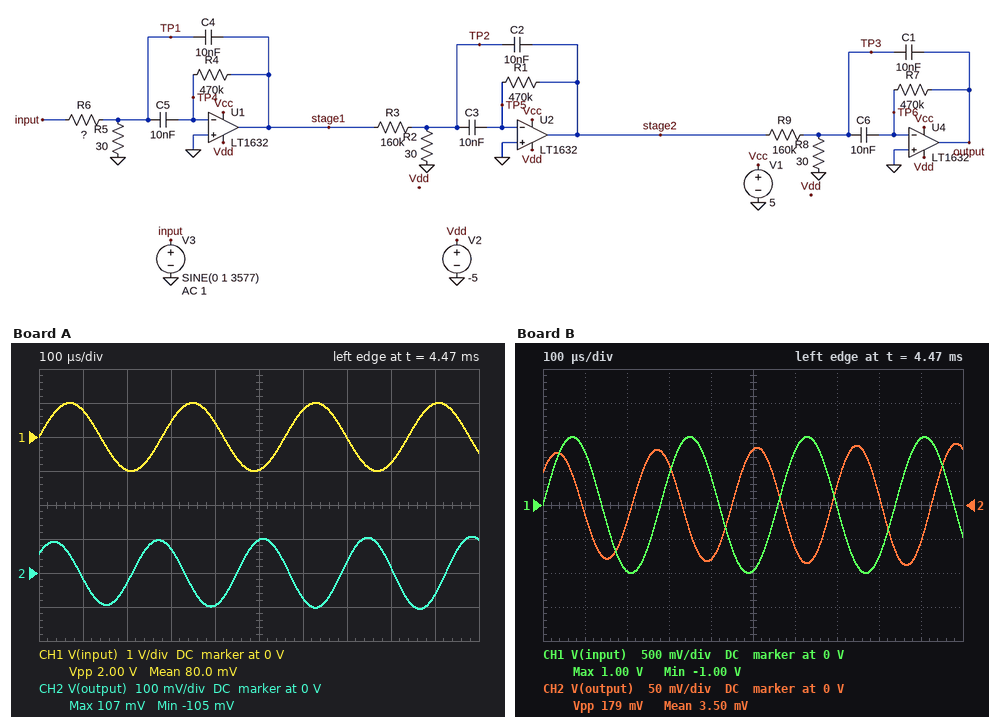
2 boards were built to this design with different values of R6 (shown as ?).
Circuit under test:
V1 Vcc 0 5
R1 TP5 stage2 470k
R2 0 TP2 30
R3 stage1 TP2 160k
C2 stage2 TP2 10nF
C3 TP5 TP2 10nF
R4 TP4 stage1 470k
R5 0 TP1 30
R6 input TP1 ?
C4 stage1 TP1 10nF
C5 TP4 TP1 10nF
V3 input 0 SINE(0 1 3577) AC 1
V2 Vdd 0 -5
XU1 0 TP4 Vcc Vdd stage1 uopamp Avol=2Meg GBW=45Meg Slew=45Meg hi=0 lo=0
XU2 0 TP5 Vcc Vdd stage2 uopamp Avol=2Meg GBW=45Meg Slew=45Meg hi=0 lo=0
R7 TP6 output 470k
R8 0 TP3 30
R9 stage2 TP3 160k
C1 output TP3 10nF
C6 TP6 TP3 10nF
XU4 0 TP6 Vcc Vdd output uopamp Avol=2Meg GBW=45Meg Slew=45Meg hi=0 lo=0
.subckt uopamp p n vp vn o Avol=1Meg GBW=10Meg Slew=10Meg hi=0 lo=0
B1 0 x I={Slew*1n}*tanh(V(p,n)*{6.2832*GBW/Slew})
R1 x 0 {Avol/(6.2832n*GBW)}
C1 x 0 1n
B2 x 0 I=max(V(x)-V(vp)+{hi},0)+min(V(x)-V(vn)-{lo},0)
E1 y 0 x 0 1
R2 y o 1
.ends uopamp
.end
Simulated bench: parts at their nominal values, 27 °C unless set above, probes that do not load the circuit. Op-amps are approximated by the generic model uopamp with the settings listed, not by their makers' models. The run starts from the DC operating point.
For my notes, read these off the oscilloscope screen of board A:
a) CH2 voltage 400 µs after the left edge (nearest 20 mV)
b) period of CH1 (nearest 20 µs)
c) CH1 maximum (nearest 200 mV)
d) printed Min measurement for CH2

-100 mV
280 µs
1.0 V
-105 mV
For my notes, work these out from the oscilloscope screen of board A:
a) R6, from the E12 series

47 kΩ
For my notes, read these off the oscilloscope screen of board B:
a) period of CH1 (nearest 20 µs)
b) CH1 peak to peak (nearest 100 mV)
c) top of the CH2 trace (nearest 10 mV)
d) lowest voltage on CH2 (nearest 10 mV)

280 µs
2.0 V
90 mV
-90 mV
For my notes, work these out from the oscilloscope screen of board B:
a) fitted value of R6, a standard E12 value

56 kΩ
